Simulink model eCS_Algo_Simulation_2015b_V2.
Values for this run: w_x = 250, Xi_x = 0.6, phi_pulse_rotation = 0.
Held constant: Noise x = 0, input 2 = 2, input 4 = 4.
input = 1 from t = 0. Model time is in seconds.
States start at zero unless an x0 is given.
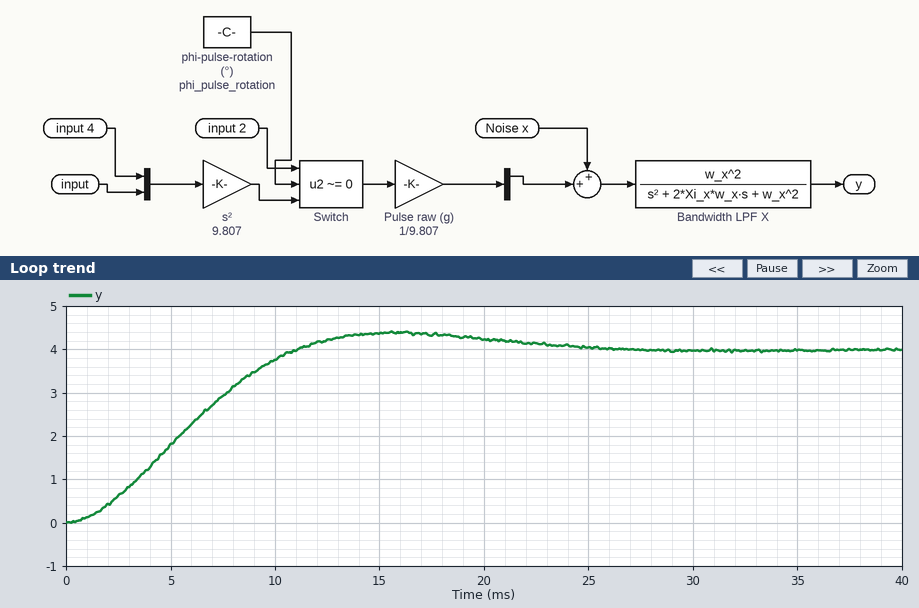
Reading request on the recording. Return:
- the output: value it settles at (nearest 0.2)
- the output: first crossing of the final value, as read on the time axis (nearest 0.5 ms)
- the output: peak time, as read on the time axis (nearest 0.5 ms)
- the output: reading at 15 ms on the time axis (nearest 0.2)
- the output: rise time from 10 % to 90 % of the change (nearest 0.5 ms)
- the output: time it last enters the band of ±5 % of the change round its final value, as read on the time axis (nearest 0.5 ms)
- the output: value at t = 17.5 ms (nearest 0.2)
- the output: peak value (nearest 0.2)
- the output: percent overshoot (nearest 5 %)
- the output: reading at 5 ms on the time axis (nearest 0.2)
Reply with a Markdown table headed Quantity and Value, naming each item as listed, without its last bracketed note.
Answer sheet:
| Quantity | Value |
|---|---|
| the output: value it settles at | 4.0 |
| the output: first crossing of the final value, as read on the time axis | 11.0 ms |
| the output: peak time, as read on the time axis | 15.5 ms |
| the output: reading at 15 ms on the time axis | 4.4 |
| the output: rise time from 10 % to 90 % of the change | 7.5 ms |
| the output: time it last enters the band of ±5 % of the change round its final value, as read on the time axis | 21.0 ms |
| the output: value at t = 17.5 ms | 4.4 |
| the output: peak value | 4.4 |
| the output: percent overshoot | 10 % |
| the output: reading at 5 ms on the time axis | 1.8 |
